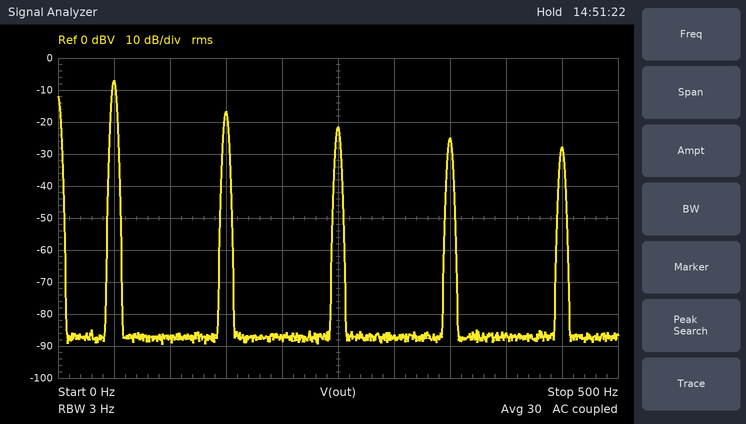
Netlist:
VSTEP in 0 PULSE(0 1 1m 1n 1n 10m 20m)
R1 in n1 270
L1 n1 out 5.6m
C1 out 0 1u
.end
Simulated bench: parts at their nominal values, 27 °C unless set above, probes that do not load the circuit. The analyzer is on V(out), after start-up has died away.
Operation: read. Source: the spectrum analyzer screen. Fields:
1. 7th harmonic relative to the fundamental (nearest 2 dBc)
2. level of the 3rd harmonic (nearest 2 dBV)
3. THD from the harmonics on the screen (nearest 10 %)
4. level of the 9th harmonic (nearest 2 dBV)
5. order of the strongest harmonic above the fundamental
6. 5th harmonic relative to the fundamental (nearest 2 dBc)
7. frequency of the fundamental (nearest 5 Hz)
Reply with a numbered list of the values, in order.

1. -18 dBc
2. -16 dBV
3. 40 %
4. -28 dBV
5. 3
6. -14 dBc
7. 50 Hz
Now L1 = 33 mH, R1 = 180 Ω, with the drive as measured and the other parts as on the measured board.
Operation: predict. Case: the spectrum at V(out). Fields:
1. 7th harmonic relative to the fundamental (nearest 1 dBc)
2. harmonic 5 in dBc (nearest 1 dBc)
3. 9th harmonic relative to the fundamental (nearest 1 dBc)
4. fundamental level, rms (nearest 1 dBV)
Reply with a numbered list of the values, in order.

1. -16 dBc
2. -14 dBc
3. -18 dBc
4. -7 dBV
